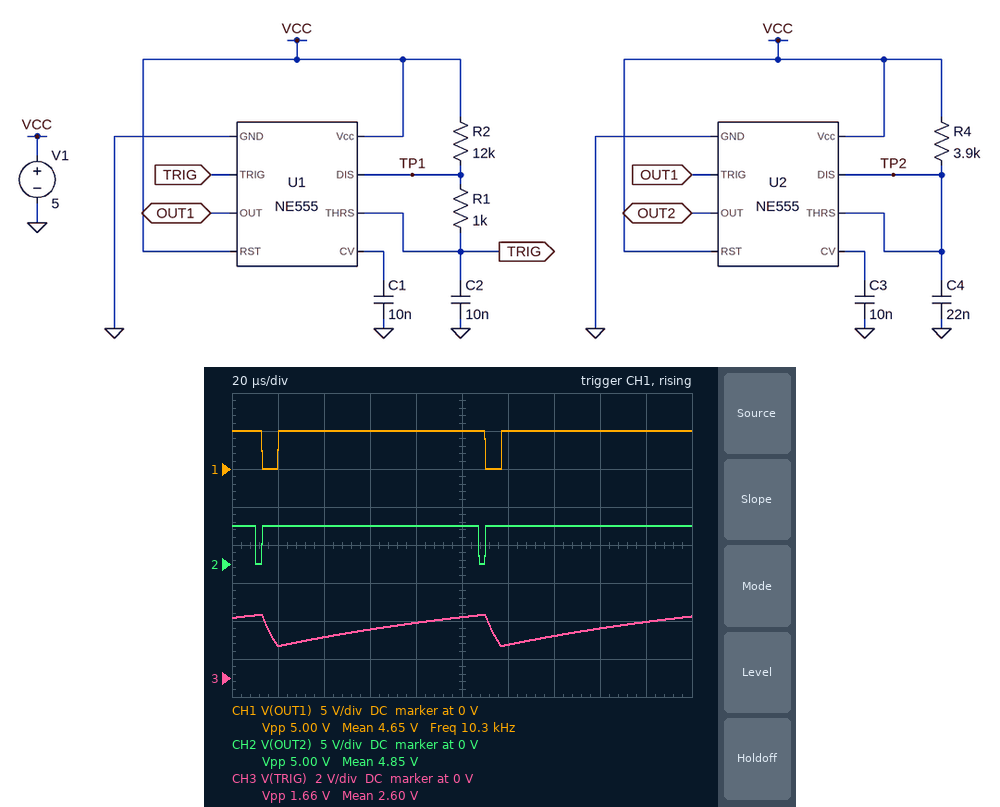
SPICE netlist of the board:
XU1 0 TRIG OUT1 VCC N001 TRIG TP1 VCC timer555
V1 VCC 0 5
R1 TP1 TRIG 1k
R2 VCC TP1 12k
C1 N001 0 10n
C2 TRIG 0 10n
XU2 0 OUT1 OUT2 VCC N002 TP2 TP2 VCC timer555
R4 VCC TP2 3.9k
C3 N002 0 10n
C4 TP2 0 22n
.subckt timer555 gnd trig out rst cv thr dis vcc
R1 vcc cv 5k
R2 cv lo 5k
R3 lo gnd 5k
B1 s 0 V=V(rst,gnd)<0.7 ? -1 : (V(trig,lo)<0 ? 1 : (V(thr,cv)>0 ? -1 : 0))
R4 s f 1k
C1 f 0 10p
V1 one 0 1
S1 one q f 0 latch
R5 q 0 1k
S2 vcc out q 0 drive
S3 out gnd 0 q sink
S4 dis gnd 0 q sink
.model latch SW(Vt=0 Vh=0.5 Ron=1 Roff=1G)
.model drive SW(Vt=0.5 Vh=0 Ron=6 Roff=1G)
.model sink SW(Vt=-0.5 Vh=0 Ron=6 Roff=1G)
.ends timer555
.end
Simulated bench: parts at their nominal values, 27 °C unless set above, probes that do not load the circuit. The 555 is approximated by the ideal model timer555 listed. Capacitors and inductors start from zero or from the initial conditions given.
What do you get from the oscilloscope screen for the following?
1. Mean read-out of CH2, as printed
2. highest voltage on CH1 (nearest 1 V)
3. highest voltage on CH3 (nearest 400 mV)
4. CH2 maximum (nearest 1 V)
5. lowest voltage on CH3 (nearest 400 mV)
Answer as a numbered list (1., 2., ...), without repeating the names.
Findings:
1. 4.85 V
2. 5 V
3. 3.2 V
4. 5 V
5. 1.6 V
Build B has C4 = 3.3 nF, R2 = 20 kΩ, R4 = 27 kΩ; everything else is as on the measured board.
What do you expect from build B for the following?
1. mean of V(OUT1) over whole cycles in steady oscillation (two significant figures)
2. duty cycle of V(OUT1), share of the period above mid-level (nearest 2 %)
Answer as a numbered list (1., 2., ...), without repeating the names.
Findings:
1. 4.8 V
2. 96 %
